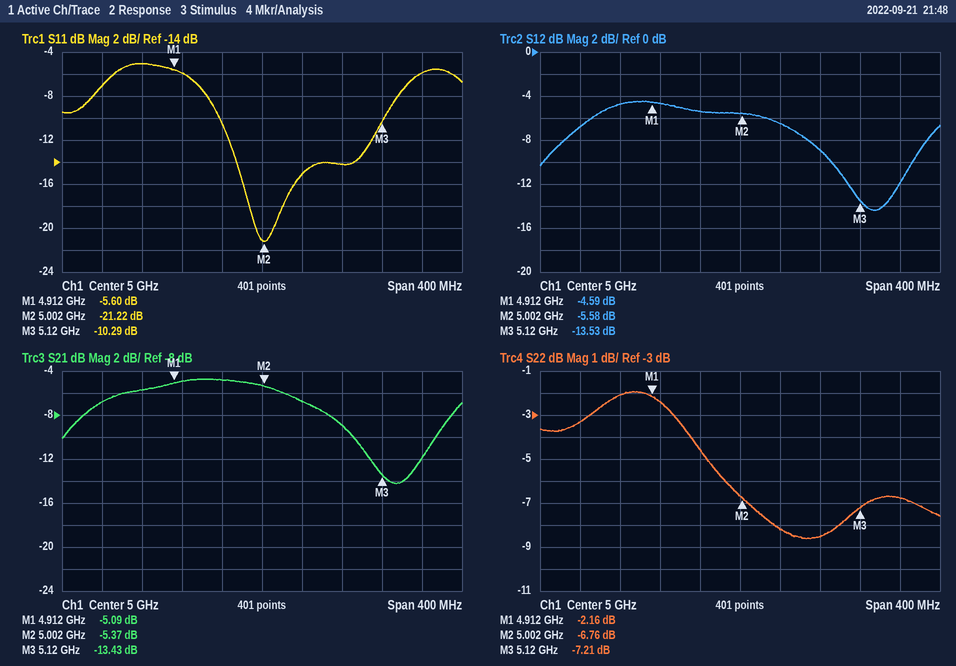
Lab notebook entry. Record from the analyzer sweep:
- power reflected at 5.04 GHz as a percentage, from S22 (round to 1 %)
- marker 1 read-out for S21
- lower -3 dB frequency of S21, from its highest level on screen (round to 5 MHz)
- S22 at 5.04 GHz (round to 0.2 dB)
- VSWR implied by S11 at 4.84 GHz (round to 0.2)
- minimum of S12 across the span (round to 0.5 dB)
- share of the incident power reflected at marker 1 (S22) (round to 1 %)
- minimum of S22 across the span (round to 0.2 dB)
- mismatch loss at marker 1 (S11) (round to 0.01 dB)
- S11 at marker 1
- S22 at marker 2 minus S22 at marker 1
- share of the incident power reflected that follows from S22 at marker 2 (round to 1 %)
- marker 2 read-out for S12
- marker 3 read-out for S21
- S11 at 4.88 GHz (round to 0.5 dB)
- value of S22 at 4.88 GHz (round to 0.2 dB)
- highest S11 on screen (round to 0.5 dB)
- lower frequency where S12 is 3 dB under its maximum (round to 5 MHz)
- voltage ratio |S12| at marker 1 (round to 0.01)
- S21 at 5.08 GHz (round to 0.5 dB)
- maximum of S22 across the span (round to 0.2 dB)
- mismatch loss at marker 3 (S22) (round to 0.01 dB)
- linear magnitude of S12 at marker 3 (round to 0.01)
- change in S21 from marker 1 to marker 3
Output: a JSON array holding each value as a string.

["15 %", "-5.09 dB", "4.825 GHz", "-8.2 dB", "2.6", "-14.5 dB", "61 %", "-8.6 dB", "1.40 dB", "-5.60 dB", "-4.60 dB", "21 %", "-5.58 dB", "-13.43 dB", "-5.0 dB", "-2.0 dB", "-5.0 dB", "4.830 GHz", "0.59", "-9.0 dB", "-2.0 dB", "0.92 dB", "0.21", "-8.34 dB"]
